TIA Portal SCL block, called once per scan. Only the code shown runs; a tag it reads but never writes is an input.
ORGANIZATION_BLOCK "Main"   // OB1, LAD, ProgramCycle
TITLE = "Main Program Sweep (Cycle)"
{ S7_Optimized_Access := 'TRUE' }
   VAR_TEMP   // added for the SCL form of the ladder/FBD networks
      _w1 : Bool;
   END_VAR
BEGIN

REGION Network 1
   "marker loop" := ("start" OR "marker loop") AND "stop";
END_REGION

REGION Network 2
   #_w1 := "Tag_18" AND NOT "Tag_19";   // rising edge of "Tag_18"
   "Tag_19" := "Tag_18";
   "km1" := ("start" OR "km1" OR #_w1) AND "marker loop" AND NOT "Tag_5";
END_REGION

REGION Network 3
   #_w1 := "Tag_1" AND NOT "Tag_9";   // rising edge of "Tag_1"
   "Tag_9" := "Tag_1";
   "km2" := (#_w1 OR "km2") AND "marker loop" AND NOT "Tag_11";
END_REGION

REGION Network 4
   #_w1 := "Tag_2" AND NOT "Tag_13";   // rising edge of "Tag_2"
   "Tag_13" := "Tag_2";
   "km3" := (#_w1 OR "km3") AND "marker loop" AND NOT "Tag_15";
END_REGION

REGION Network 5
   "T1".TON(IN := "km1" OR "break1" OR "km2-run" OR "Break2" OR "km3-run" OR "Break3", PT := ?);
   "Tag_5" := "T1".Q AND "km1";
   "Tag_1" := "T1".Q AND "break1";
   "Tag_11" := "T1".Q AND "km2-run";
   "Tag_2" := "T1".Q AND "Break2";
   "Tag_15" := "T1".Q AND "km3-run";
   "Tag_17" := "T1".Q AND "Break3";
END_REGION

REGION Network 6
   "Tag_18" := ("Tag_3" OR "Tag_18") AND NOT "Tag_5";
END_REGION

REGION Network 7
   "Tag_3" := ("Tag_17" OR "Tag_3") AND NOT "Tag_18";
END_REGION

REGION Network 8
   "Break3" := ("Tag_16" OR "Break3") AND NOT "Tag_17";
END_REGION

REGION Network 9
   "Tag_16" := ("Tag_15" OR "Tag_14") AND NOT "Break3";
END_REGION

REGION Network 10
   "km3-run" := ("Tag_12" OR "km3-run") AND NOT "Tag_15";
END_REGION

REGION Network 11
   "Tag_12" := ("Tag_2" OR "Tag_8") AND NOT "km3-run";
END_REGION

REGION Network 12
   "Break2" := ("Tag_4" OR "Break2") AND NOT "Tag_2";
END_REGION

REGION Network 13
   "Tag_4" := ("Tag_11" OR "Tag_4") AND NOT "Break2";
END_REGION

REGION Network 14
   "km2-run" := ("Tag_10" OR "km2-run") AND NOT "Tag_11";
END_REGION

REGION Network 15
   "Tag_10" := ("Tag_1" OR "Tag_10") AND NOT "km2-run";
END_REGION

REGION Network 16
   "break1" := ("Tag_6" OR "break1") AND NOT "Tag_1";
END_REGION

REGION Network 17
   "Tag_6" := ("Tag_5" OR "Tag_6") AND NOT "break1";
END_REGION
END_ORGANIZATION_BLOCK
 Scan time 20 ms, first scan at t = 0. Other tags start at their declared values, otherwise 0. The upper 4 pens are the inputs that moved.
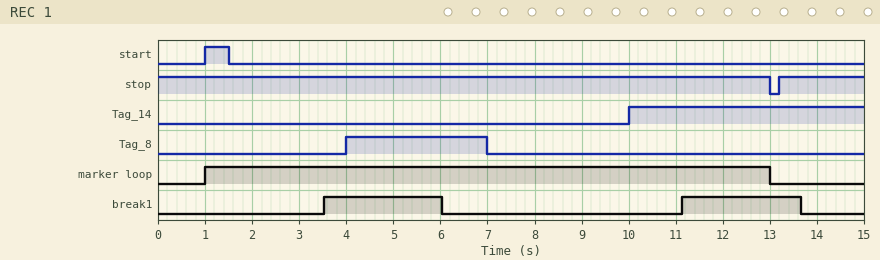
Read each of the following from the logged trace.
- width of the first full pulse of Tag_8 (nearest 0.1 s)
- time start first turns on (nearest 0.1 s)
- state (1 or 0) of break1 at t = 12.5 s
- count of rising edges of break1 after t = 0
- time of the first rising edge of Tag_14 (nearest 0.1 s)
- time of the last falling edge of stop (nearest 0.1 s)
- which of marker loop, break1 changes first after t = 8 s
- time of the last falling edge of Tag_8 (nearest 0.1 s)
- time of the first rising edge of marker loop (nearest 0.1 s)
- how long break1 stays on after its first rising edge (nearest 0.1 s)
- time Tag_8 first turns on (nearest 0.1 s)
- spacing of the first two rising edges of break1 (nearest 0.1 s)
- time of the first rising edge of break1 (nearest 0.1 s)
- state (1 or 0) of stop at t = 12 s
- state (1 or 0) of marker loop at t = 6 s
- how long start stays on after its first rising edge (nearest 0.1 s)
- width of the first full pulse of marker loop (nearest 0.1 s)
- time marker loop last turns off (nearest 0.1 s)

3.0 s
1.0 s
1
2
10.0 s
13.0 s
break1
7.0 s
1.0 s
2.5 s
4.0 s
7.6 s
3.5 s
1
1
0.5 s
12.0 s
13.0 s
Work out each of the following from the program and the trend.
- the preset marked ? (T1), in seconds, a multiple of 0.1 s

2.5 s
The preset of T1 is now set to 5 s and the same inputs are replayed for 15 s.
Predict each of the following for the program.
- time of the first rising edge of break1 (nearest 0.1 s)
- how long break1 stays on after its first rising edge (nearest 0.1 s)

6.0 s
5.0 s
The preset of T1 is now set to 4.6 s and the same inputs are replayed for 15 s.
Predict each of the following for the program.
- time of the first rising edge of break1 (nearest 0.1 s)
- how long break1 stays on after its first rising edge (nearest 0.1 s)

5.6 s
4.6 s
